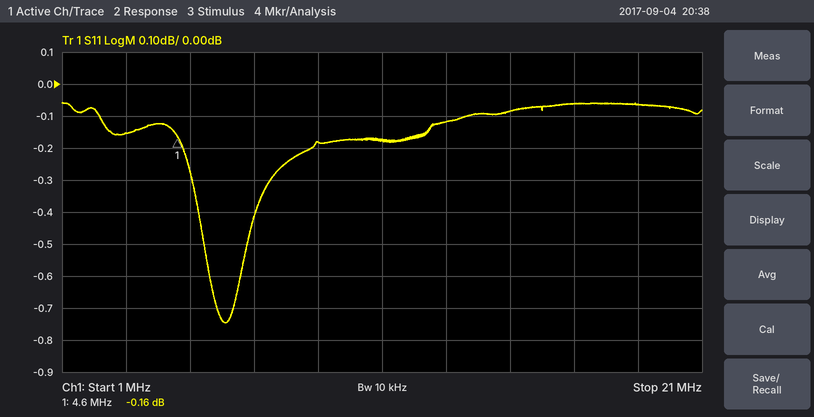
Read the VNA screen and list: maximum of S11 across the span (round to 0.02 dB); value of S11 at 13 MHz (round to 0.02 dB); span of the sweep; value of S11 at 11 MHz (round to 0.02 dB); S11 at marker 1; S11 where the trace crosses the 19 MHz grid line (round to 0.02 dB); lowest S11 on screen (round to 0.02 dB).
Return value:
-0.06 dB
-0.12 dB
20 MHz
-0.18 dB
-0.16 dB
-0.06 dB
-0.74 dB
